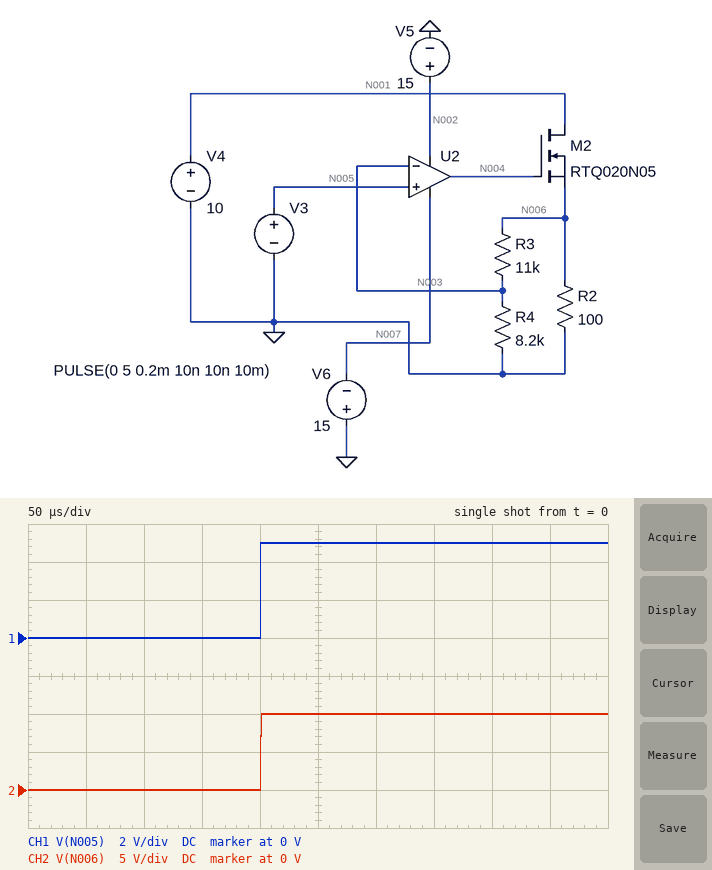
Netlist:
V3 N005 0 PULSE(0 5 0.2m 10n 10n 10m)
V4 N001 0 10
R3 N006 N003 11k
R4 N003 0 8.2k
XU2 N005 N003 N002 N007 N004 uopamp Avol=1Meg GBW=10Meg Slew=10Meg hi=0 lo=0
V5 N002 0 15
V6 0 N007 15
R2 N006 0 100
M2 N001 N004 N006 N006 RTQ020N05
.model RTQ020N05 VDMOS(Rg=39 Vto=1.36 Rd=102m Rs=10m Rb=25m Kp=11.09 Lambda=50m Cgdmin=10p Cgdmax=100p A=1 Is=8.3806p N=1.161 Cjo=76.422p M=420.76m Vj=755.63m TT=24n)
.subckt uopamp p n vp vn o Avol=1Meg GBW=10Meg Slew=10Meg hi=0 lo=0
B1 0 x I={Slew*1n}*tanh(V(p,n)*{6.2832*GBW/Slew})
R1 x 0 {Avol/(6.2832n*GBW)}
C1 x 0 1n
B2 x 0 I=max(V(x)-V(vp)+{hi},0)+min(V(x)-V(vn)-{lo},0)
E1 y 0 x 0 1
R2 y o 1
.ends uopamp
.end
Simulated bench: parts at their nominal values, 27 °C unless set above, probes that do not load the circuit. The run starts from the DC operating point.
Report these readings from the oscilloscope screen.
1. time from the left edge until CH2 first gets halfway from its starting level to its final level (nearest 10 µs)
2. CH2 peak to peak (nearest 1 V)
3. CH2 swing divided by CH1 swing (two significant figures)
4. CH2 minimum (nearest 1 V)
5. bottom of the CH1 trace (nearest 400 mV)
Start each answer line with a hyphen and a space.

- 200 µs
- 10 V
- 2.0
- 0 V
- 0 V
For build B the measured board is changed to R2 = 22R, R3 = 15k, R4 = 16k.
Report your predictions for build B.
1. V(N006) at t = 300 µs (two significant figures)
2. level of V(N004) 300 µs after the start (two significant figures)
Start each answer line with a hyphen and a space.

- 9.7 V
- 11 V
